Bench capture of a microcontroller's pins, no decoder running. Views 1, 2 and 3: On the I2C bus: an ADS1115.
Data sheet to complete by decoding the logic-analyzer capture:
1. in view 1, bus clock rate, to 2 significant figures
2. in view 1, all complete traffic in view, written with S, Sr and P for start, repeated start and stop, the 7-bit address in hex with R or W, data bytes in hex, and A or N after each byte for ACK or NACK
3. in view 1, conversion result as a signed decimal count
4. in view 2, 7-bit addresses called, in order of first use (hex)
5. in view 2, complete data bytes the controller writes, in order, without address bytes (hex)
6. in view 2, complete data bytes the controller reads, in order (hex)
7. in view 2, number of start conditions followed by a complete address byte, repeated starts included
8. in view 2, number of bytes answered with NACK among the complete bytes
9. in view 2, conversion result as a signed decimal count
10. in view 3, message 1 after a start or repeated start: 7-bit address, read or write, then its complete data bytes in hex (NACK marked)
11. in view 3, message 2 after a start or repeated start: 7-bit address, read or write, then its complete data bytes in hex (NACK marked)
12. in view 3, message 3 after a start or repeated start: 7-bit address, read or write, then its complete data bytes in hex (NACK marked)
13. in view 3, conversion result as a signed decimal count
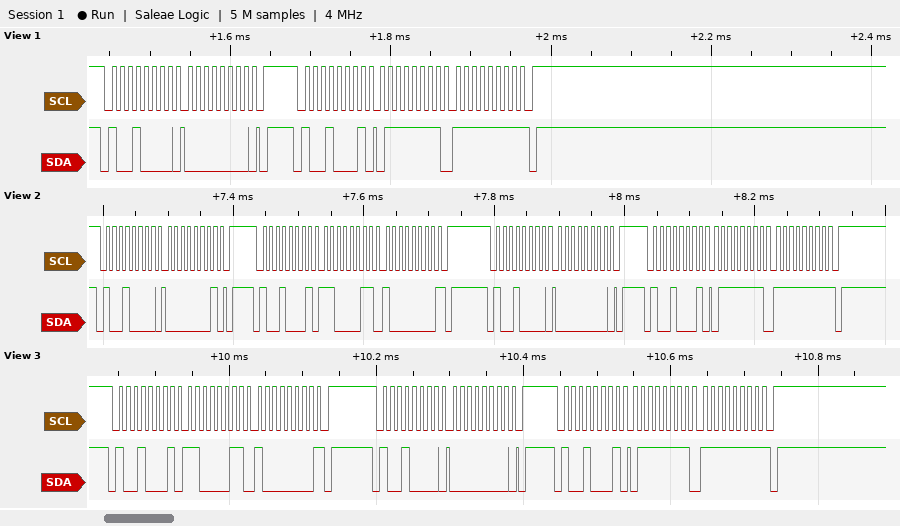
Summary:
100 kHz
S 48W A 00 A P S 48R A 7F A FF N P
32767
0x48
01 00
C3 80 7F FF
4
2
32767
0x48 read: C3 80 NACK
0x48 write: 00
0x48 read: 7F FF NACK
32767
